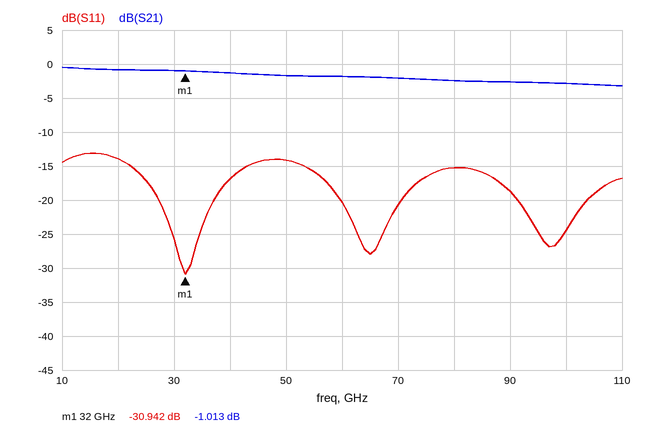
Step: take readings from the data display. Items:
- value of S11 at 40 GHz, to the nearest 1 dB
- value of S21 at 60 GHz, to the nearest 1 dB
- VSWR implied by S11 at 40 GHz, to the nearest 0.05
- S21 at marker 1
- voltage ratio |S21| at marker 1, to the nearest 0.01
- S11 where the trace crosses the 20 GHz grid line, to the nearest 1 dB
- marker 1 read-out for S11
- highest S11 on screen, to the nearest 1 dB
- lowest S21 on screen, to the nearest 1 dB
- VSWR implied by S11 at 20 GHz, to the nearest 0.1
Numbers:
-17 dB
-2 dB
1.35
-1.013 dB
0.89
-14 dB
-30.942 dB
-13 dB
-3 dB
1.5
